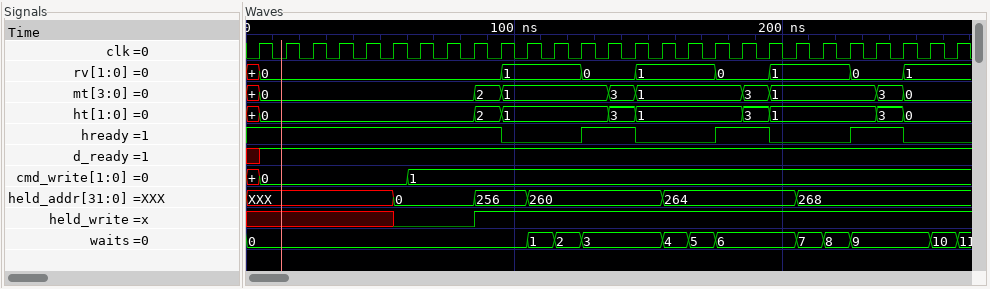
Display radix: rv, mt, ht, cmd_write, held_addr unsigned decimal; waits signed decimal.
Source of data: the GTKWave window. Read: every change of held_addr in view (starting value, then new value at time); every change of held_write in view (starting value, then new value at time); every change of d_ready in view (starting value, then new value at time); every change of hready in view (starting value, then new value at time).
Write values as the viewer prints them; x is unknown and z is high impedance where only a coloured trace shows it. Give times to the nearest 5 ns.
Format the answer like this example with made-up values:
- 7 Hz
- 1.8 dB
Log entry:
- XXX, 0 at 55 ns, 256 at 85 ns, 260 at 105 ns, 264 at 155 ns, 268 at 205 ns
- x, 0 at 55 ns, 1 at 85 ns
- x, 1 at 5 ns
- 1, 0 at 95 ns, 1 at 125 ns, 0 at 145 ns, 1 at 175 ns, 0 at 195 ns, 1 at 225 ns, 0 at 245 ns
